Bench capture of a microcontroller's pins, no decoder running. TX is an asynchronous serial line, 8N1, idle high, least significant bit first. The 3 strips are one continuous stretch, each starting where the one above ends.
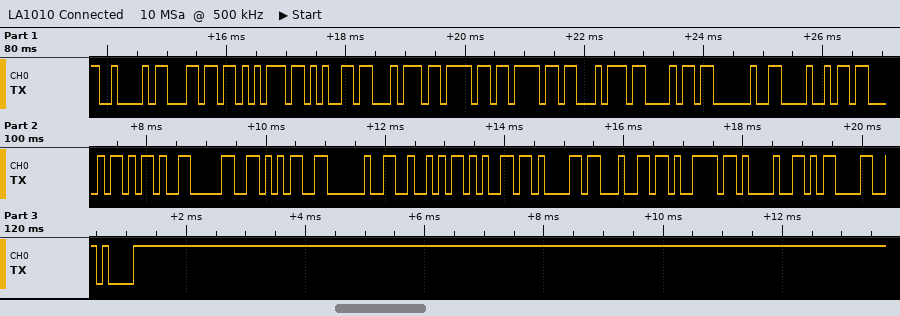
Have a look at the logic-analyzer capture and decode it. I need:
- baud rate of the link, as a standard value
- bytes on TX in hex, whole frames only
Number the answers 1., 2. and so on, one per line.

1. 9600 baud
2. 42 6C 75 65 74 6F 6F 74 68 20 48 43 2D 30 35 20 52 65 61 64 79 21 0D 0A
